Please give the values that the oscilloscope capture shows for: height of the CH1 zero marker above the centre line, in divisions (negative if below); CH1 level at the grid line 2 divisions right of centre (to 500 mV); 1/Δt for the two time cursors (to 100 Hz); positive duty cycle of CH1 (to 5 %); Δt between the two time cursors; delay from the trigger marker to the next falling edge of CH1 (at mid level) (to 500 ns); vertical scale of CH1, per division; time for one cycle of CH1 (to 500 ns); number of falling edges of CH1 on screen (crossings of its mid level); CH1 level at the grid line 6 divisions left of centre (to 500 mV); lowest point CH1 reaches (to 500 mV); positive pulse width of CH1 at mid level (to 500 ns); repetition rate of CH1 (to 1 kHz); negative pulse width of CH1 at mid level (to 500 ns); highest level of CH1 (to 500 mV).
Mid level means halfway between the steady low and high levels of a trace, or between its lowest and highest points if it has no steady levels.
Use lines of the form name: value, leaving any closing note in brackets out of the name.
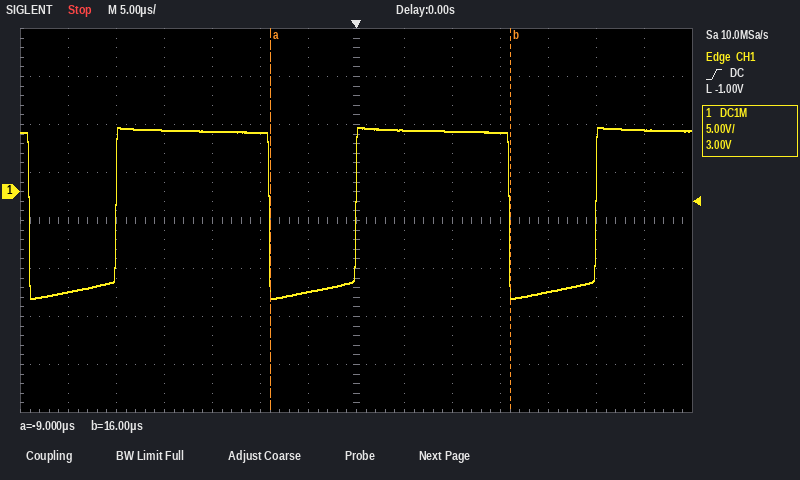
height of the CH1 zero marker above the centre line, in divisions: +0.6 div
CH1 level at the grid line 2 divisions right of centre: 6.5 V
1/Δt for the two time cursors: 40.0 kHz
positive duty cycle of CH1: 65 %
Δt between the two time cursors: 25.0 µs
delay from the trigger marker to the next falling edge of CH1 (at mid level): 16.0 µs
vertical scale of CH1, per division: 5 V
time for one cycle of CH1: 25.0 µs
number of falling edges of CH1 on screen: 3
CH1 level at the grid line 6 divisions left of centre: -10.5 V
lowest point CH1 reaches: -11.0 V
positive pulse width of CH1 at mid level: 16.0 µs
repetition rate of CH1: 40 kHz
negative pulse width of CH1 at mid level: 9.0 µs
highest level of CH1: 6.5 V
